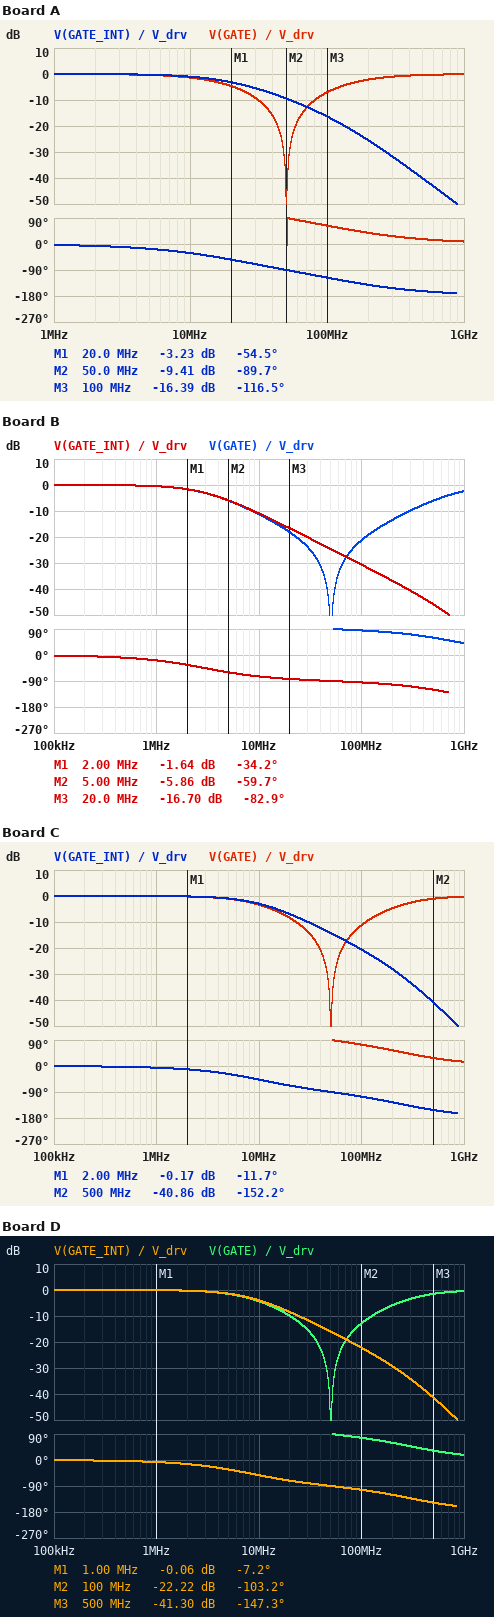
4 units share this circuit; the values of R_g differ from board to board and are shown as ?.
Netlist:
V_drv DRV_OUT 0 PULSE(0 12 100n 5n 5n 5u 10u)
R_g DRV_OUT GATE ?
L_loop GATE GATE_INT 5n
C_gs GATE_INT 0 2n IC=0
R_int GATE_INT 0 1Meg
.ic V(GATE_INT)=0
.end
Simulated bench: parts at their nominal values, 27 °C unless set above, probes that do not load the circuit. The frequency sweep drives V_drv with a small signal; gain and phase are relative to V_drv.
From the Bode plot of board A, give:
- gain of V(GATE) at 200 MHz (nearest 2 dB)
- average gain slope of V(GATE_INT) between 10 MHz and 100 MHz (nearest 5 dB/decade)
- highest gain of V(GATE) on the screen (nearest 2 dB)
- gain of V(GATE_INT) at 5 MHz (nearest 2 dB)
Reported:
-2 dB
-15 dB/decade
0 dB
0 dB
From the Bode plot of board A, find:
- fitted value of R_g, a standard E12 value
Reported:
4.7 Ω
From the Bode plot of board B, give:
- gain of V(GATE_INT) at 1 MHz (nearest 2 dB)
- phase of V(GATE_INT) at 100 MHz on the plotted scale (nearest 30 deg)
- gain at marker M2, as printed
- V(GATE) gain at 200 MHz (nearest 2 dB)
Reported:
0 dB
-90 deg
-5.86 dB
-14 dB
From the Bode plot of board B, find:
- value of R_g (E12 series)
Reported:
27 Ω
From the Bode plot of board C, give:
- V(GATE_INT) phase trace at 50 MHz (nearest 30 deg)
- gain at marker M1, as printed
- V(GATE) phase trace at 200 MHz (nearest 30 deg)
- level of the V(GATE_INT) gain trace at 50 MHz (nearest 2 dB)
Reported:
-90 deg
-0.17 dB
60 deg
-14 dB
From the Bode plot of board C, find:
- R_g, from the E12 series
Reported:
8.2 Ω
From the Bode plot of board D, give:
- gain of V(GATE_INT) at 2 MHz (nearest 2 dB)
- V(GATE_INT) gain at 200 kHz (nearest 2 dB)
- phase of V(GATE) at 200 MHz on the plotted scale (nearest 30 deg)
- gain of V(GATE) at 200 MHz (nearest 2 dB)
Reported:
0 dB
0 dB
60 deg
-6 dB
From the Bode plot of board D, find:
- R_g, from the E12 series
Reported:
10 Ω
